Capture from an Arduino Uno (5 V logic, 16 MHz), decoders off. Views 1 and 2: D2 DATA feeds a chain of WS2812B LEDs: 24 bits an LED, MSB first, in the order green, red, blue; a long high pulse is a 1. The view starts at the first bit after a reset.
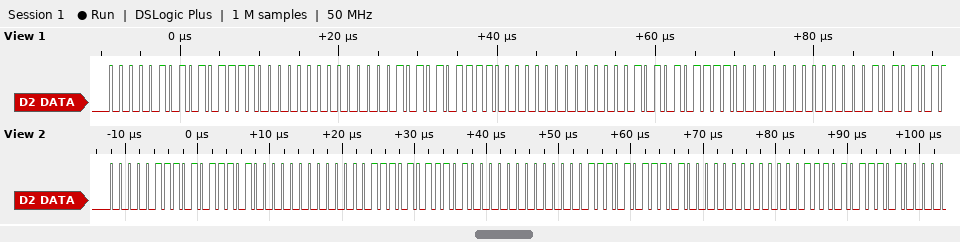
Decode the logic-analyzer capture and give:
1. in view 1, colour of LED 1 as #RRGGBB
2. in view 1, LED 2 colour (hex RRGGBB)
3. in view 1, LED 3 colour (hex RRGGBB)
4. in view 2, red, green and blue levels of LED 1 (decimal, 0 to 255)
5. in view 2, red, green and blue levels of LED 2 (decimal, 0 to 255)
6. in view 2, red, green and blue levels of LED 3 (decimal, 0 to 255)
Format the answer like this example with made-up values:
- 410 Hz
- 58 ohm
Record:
- #5E0500
- #5E0500
- #5E0500
- 93, 7, 0
- 93, 7, 0
- 93, 7, 0
